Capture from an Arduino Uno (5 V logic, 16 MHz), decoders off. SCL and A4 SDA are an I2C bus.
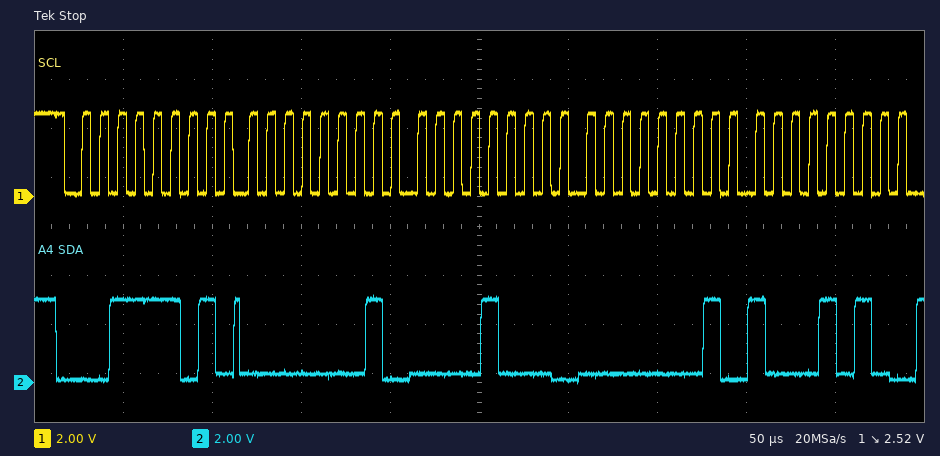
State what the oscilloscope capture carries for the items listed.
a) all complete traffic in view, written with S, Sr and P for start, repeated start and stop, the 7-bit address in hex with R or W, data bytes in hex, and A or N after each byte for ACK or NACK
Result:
S 1ER A 01 A 08 A 01 A 8A A
